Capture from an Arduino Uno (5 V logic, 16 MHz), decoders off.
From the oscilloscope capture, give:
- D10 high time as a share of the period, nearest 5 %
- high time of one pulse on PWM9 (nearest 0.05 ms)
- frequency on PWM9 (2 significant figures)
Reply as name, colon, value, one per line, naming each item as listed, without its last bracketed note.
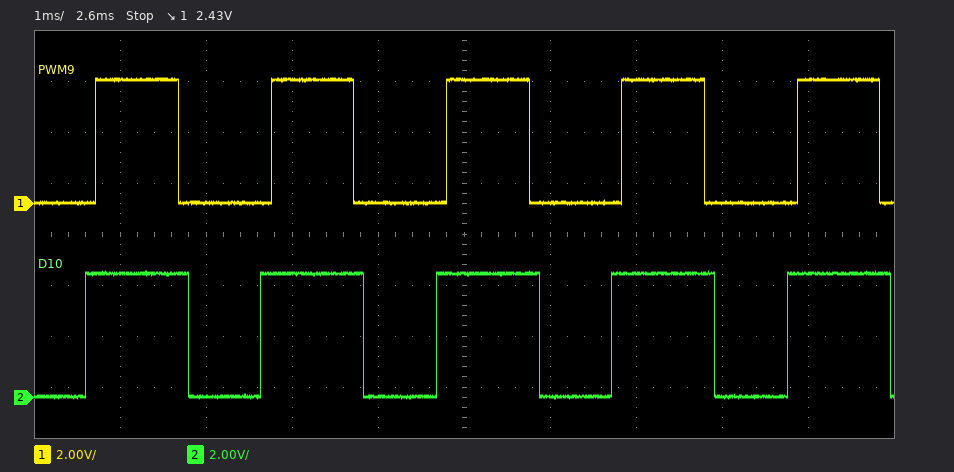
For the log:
D10 high time as a share of the period, nearest 5 %: 60 %
high time of one pulse on PWM9: 0.95 ms
frequency on PWM9: 490 Hz
